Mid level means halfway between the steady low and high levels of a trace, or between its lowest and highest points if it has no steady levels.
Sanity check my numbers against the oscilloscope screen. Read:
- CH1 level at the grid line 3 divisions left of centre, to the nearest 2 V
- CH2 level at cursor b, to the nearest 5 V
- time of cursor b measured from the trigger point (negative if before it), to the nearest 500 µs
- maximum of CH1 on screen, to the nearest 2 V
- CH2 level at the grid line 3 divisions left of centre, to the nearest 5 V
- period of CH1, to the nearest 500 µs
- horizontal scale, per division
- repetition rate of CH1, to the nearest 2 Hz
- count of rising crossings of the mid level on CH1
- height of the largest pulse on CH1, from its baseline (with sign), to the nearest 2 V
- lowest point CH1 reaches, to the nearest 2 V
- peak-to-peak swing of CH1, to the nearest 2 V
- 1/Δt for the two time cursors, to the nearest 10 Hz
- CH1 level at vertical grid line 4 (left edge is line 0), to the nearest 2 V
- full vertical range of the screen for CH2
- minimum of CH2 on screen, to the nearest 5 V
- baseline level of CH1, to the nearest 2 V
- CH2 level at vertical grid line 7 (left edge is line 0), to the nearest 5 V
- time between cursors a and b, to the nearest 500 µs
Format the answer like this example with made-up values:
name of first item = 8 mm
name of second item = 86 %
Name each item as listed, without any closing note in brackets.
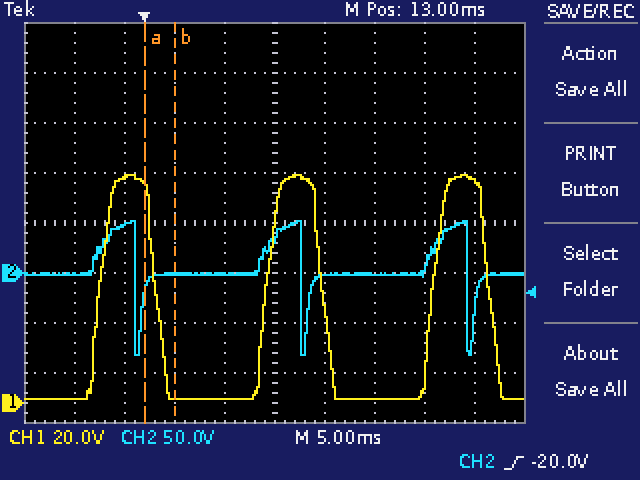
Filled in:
CH1 level at the grid line 3 divisions left of centre, to the nearest 2 V = 90 V
CH2 level at cursor b, to the nearest 5 V = 0 V
time of cursor b measured from the trigger point (negative if before it), to the nearest 500 µs = +3.0 ms
maximum of CH1 on screen, to the nearest 2 V = 92 V
CH2 level at the grid line 3 divisions left of centre, to the nearest 5 V = 50 V
period of CH1, to the nearest 500 µs = 16.5 ms
horizontal scale, per division = 5 ms
repetition rate of CH1, to the nearest 2 Hz = 60 Hz
count of rising crossings of the mid level on CH1 = 3
height of the largest pulse on CH1, from its baseline (with sign), to the nearest 2 V = +90 V
lowest point CH1 reaches, to the nearest 2 V = 2 V
peak-to-peak swing of CH1, to the nearest 2 V = 90 V
1/Δt for the two time cursors, to the nearest 10 Hz = 330 Hz
CH1 level at vertical grid line 4 (left edge is line 0), to the nearest 2 V = 2 V
full vertical range of the screen for CH2 = 400 V
minimum of CH2 on screen, to the nearest 5 V = -80 V
baseline level of CH1, to the nearest 2 V = 2 V
CH2 level at vertical grid line 7 (left edge is line 0), to the nearest 5 V = 0 V
time between cursors a and b, to the nearest 500 µs = 3.0 ms
